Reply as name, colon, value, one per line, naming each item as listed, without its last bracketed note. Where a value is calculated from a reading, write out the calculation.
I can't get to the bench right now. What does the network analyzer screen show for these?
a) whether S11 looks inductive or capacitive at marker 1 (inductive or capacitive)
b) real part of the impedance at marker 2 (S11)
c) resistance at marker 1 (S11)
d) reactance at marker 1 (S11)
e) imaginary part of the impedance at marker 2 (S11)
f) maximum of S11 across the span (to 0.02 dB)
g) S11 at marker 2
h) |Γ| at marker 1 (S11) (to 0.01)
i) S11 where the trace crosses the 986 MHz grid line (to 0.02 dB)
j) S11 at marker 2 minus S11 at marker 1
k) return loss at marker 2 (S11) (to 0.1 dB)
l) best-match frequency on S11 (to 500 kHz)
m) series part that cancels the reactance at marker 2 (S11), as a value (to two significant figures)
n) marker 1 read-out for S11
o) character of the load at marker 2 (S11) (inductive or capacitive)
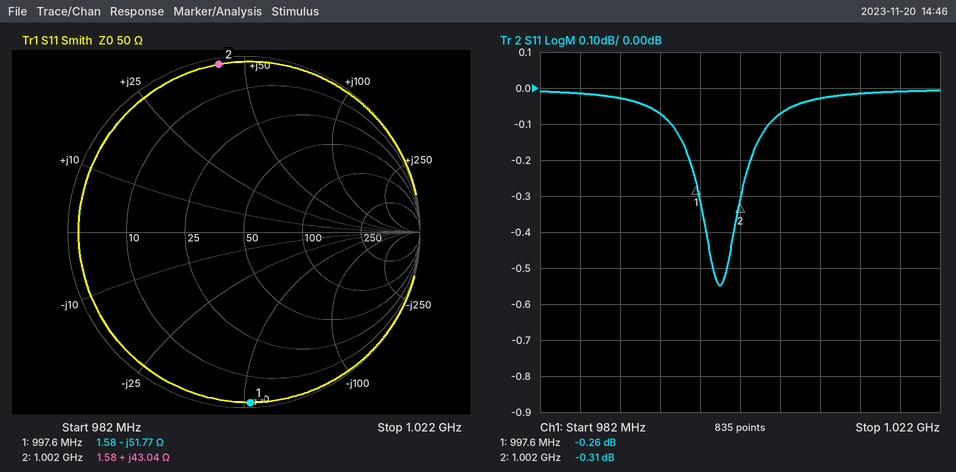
whether S11 looks inductive or capacitive at marker 1: capacitive
real part of the impedance at marker 2: 1.58 Ω
resistance at marker 1: 1.58 Ω
reactance at marker 1: -51.77 Ω
imaginary part of the impedance at marker 2: +43.04 Ω
maximum of S11 across the span: 0.00 dB
S11 at marker 2: -0.31 dB
|Γ| at marker 1 (S11): 0.97
S11 where the trace crosses the 986 MHz grid line: -0.02 dB
S11 at marker 2 minus S11 at marker 1: -0.31 − (-0.26) = -0.05 dB
return loss at marker 2 (S11): 0.3 dB
best-match frequency on S11: 1.0000 GHz
series part that cancels the reactance at marker 2 (S11), as a value: C = 1/(2π × 1.002 GHz × 43.04 Ω) ≈ 3.7 pF
marker 1 read-out for S11: -0.26 dB
character of the load at marker 2 (S11): inductive
